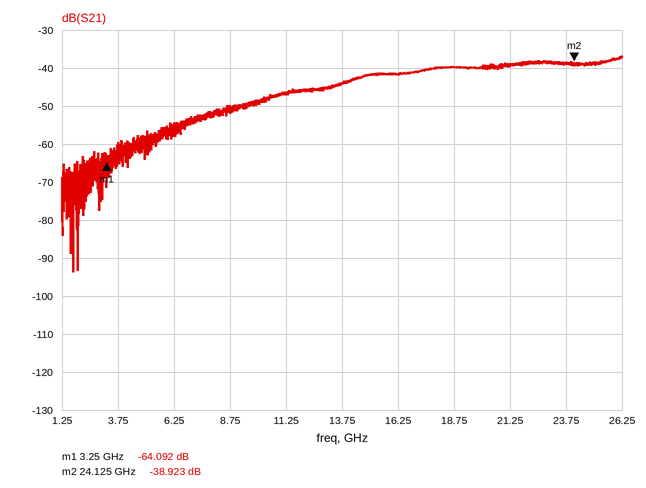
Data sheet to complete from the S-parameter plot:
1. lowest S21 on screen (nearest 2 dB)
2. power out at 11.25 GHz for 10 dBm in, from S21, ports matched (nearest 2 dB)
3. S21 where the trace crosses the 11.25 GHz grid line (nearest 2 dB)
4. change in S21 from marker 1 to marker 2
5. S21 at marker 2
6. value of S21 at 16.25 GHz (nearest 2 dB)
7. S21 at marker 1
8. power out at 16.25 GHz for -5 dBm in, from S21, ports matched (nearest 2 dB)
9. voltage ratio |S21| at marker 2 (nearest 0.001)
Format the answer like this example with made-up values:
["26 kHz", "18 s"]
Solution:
["-94 dB", "-36 dBm", "-46 dB", "25.169 dB", "-38.923 dB", "-42 dB", "-64.092 dB", "-46 dBm", "0.011"]
